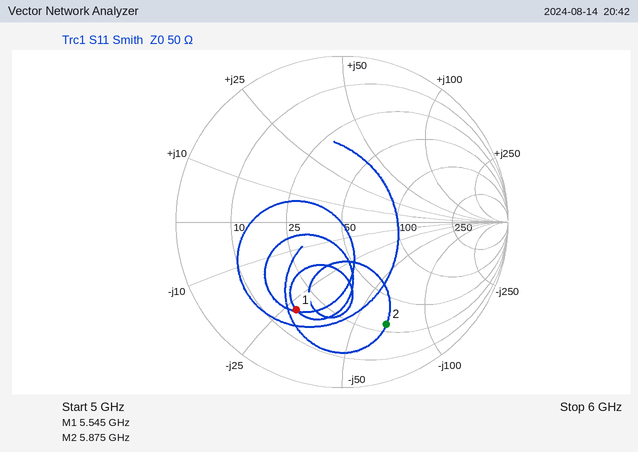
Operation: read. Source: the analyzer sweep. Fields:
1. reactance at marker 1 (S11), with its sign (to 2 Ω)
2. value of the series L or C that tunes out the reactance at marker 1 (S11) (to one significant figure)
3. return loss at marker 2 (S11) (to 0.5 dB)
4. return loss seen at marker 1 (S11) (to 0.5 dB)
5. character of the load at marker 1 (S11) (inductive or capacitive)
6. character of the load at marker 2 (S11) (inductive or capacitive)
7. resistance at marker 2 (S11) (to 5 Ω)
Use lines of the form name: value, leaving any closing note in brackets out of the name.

reactance at marker 1 (S11), with its sign: -28 Ω
value of the series L or C that tunes out the reactance at marker 1 (S11): 800 pH
return loss at marker 2 (S11): 3.5 dB
return loss seen at marker 1 (S11): 4.5 dB
character of the load at marker 1 (S11): capacitive
character of the load at marker 2 (S11): capacitive
resistance at marker 2 (S11): 30 Ω
